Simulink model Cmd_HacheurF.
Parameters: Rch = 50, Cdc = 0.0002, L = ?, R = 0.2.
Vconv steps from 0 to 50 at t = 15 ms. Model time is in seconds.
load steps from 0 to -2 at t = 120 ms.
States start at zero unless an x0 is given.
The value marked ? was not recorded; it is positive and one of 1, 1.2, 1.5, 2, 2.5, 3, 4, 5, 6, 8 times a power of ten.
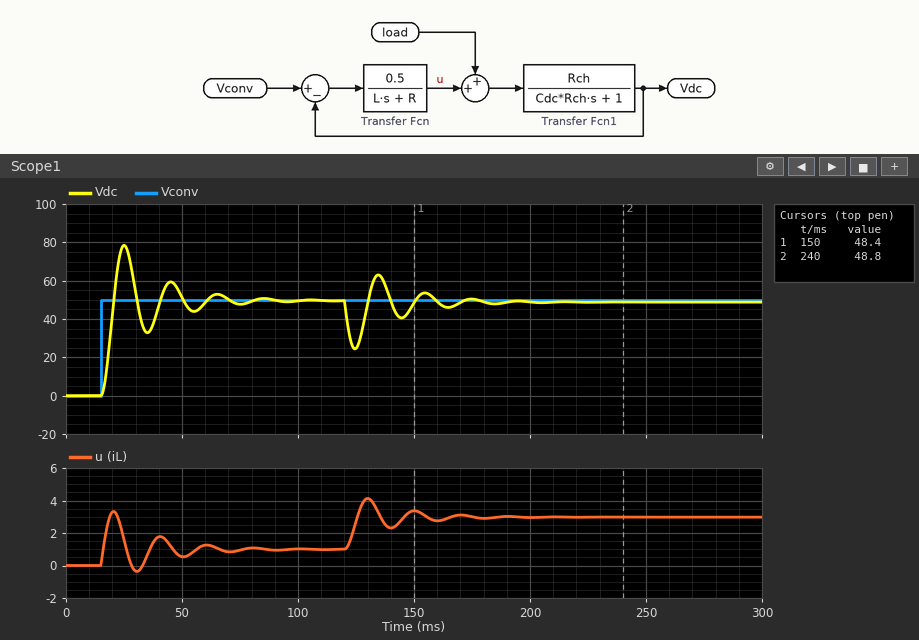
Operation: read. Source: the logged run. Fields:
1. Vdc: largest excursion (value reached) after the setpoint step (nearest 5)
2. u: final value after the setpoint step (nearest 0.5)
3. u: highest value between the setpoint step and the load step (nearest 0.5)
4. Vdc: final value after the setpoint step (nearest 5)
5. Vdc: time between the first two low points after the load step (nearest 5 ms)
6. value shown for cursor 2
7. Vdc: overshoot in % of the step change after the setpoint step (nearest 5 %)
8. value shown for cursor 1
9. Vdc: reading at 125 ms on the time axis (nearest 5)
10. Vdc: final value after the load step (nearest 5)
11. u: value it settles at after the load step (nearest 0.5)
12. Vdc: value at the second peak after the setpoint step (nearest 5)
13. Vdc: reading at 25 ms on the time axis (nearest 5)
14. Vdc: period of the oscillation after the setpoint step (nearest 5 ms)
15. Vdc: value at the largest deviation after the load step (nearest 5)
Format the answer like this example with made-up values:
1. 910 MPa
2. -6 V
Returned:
1. 80
2. 1.0
3. 3.5
4. 50
5. 20 ms
6. 48.8
7. 60 %
8. 48.4
9. 25
10. 50
11. 3.0
12. 60
13. 80
14. 20 ms
15. 25
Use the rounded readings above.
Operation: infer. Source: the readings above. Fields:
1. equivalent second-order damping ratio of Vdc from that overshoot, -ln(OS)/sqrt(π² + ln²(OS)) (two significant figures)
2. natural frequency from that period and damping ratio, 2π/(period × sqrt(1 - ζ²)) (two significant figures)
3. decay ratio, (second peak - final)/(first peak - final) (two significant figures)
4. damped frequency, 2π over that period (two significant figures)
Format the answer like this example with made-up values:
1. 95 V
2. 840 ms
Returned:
1. 0.16
2. 0.32 rad/ms
3. 0.33
4. 0.31 rad/ms
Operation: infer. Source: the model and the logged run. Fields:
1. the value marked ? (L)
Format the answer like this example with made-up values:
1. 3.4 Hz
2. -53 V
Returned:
1. 0.025
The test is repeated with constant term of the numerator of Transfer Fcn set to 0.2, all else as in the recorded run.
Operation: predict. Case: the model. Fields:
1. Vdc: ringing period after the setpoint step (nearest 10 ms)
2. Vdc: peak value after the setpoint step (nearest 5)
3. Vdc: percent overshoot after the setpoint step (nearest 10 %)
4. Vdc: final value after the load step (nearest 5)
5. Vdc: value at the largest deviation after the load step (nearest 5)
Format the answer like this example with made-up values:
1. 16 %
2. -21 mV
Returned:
1. 30 ms
2. 70
3. 40 %
4. 45
5. 15
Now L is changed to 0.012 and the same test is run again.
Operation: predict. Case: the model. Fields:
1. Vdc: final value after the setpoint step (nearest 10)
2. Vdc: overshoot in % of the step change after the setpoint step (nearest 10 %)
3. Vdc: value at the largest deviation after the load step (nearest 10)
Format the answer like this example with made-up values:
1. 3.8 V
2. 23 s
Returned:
1. 50
2. 70 %
3. 30
